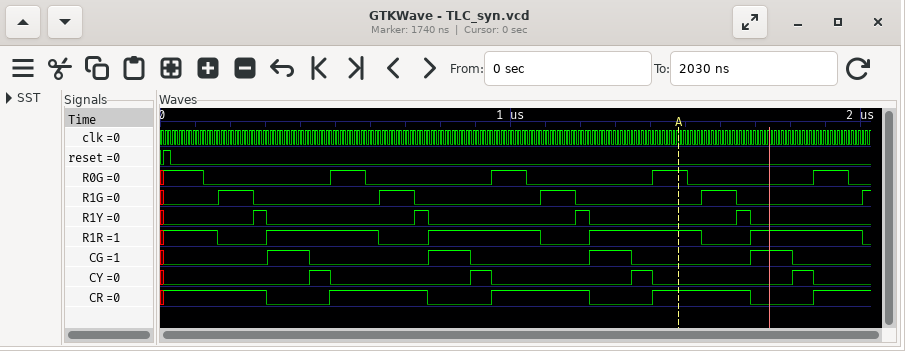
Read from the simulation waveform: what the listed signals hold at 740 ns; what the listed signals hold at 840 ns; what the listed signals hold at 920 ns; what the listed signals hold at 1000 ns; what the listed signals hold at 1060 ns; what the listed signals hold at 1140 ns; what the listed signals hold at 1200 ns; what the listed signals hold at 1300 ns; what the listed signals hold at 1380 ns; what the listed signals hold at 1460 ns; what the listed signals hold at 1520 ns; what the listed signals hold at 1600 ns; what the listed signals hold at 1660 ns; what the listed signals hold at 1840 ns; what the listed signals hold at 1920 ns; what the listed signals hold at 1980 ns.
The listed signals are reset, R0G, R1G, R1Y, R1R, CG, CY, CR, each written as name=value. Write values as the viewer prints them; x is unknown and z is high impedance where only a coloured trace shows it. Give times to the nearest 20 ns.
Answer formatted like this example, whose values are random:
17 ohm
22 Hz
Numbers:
reset=0, R0G=0, R1G=0, R1Y=1, R1R=0, CG=0, CY=0, CR=1
reset=0, R0G=0, R1G=0, R1Y=0, R1R=1, CG=1, CY=0, CR=0
reset=0, R0G=0, R1G=0, R1Y=0, R1R=1, CG=0, CY=1, CR=0
reset=0, R0G=1, R1G=0, R1Y=0, R1R=1, CG=0, CY=0, CR=1
reset=0, R0G=0, R1G=0, R1Y=0, R1R=1, CG=0, CY=0, CR=1
reset=0, R0G=0, R1G=1, R1Y=0, R1R=0, CG=0, CY=0, CR=1
reset=0, R0G=0, R1G=0, R1Y=1, R1R=0, CG=0, CY=0, CR=1
reset=0, R0G=0, R1G=0, R1Y=0, R1R=1, CG=1, CY=0, CR=0
reset=0, R0G=0, R1G=0, R1Y=0, R1R=1, CG=0, CY=1, CR=0
reset=0, R0G=1, R1G=0, R1Y=0, R1R=1, CG=0, CY=0, CR=1
reset=0, R0G=0, R1G=0, R1Y=0, R1R=1, CG=0, CY=0, CR=1
reset=0, R0G=0, R1G=1, R1Y=0, R1R=0, CG=0, CY=0, CR=1
reset=0, R0G=0, R1G=0, R1Y=1, R1R=0, CG=0, CY=0, CR=1
reset=0, R0G=0, R1G=0, R1Y=0, R1R=1, CG=0, CY=1, CR=0
reset=0, R0G=1, R1G=0, R1Y=0, R1R=1, CG=0, CY=0, CR=1
reset=0, R0G=0, R1G=0, R1Y=0, R1R=1, CG=0, CY=0, CR=1
